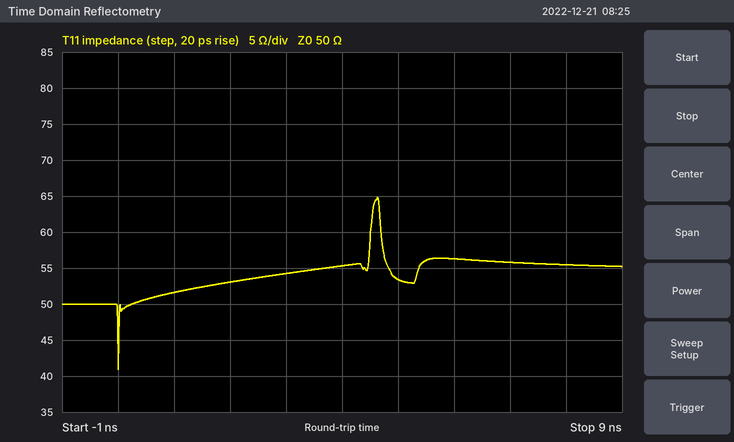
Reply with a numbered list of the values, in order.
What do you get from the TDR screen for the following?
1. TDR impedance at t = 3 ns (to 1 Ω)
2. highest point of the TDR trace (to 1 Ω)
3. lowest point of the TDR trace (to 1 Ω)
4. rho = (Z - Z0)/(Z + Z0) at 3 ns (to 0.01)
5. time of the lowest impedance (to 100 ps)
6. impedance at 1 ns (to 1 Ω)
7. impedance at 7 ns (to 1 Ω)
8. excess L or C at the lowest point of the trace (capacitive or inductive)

1. 54 Ω
2. 65 Ω
3. 41 Ω
4. +0.04
5. 0.0 ns
6. 52 Ω
7. 56 Ω
8. capacitive
